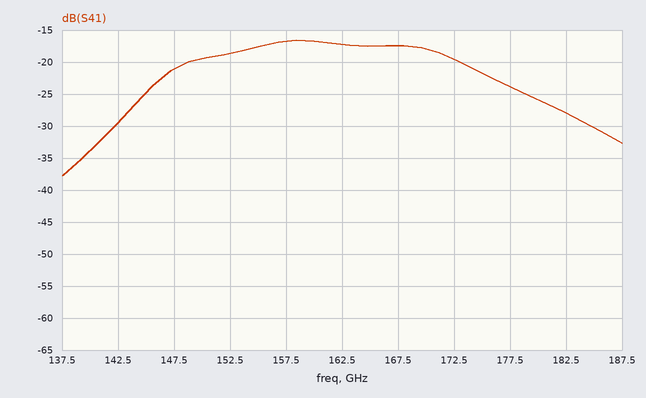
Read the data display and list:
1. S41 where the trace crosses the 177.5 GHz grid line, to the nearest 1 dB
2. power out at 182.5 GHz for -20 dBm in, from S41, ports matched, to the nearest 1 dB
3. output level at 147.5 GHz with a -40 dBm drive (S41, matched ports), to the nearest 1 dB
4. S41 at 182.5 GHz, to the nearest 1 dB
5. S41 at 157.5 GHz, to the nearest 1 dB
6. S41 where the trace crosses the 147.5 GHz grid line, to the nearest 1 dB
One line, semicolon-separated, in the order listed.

-24 dB; -48 dBm; -61 dBm; -28 dB; -17 dB; -21 dB
